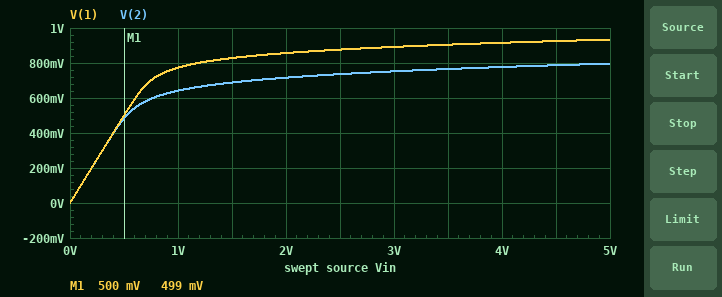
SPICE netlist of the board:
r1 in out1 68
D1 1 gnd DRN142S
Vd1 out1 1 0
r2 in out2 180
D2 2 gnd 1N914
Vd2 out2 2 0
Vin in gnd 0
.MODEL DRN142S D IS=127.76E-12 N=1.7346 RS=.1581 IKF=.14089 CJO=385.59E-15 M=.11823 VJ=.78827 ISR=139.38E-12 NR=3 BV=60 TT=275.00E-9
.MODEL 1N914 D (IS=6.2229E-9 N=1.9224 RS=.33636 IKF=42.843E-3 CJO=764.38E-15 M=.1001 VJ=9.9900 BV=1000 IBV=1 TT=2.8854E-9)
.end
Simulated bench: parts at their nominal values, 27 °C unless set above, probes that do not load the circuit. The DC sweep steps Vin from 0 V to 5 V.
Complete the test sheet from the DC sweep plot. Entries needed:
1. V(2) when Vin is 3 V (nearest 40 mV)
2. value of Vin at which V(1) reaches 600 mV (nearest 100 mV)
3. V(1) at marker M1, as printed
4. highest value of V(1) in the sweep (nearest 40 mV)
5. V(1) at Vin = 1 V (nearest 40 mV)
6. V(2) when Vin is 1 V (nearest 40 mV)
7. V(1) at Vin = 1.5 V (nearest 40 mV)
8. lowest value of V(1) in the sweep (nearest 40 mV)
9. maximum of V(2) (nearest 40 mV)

760 mV
600 mV
499 mV
920 mV
760 mV
640 mV
840 mV
0 V
800 mV
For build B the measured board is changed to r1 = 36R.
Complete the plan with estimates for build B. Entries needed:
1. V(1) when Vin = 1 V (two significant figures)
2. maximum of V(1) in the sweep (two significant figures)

800 mV
980 mV
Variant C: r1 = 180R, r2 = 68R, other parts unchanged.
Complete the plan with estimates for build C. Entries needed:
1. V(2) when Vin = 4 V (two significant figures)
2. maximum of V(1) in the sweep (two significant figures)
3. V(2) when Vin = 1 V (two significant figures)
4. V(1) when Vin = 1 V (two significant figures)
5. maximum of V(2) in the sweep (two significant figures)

850 mV
870 mV
690 mV
730 mV
880 mV
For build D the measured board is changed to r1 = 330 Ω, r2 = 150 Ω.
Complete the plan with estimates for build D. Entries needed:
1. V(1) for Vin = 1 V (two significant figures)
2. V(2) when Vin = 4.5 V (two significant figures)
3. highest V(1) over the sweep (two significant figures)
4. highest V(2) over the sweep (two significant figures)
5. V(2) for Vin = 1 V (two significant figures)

710 mV
800 mV
840 mV
810 mV
650 mV
